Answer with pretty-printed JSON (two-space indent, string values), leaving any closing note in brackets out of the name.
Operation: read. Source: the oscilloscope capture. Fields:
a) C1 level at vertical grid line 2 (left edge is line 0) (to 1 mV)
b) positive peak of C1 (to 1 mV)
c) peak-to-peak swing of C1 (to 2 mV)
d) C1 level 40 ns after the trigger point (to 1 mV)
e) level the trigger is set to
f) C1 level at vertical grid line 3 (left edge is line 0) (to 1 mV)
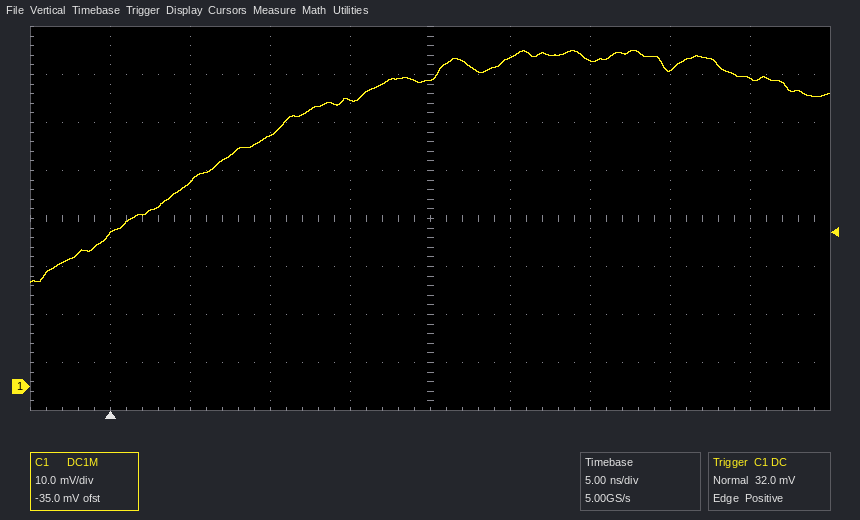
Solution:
{
  "C1 level at vertical grid line 2 (left edge is line 0)": "43 mV",
  "positive peak of C1": "70 mV",
  "peak-to-peak swing of C1": "48 mV",
  "C1 level 40 ns after the trigger point": "64 mV",
  "level the trigger is set to": "32.0 mV",
  "C1 level at vertical grid line 3 (left edge is line 0)": "52 mV"
}
